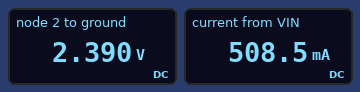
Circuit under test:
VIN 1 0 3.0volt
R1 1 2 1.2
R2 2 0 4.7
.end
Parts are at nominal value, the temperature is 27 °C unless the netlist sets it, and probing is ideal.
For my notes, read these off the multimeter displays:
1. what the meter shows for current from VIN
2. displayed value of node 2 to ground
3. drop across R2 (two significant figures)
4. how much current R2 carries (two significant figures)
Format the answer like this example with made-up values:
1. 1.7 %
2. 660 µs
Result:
1. 508.5 mA
2. 2.390 V
3. 2.4 V
4. 510 mA
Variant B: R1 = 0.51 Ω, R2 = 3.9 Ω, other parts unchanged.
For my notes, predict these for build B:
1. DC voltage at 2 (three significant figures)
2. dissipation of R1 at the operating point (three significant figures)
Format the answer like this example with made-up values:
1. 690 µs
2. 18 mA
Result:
1. 2.65 V
2. 236 mW
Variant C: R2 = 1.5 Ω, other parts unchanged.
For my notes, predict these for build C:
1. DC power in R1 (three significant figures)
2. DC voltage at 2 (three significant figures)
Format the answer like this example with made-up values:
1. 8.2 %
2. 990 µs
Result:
1. 1.48 W
2. 1.67 V
